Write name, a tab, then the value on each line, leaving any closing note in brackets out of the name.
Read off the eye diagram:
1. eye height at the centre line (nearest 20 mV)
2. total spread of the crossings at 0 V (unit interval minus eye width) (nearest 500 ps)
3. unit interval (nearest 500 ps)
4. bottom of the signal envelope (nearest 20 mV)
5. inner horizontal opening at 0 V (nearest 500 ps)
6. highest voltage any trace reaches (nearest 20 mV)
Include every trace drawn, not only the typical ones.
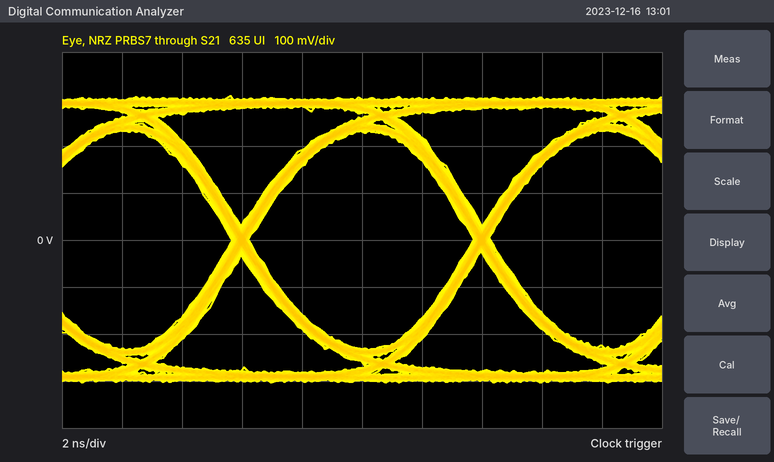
eye height at the centre line	460 mV
total spread of the crossings at 0 V (unit interval minus eye width)	500 ps
unit interval	8.0 ns
bottom of the signal envelope	-300 mV
inner horizontal opening at 0 V	7.5 ns
highest voltage any trace reaches	300 mV
